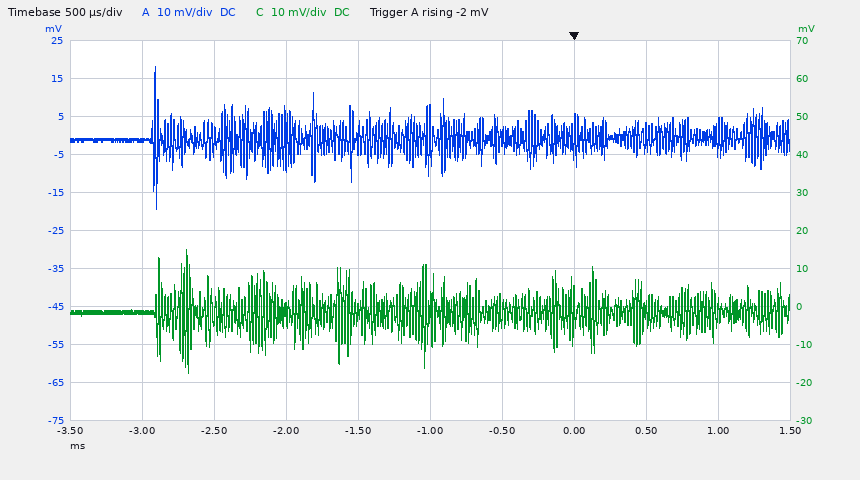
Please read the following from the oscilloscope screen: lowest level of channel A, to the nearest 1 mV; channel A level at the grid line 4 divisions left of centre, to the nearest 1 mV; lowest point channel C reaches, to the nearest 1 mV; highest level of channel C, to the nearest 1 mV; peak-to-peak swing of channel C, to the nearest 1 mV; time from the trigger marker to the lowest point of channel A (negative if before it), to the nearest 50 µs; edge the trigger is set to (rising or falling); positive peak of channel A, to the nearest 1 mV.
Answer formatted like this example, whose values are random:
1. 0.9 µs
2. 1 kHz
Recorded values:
1. -19 mV
2. -1 mV
3. -17 mV
4. 15 mV
5. 32 mV
6. -2.90 ms
7. rising
8. 18 mV
